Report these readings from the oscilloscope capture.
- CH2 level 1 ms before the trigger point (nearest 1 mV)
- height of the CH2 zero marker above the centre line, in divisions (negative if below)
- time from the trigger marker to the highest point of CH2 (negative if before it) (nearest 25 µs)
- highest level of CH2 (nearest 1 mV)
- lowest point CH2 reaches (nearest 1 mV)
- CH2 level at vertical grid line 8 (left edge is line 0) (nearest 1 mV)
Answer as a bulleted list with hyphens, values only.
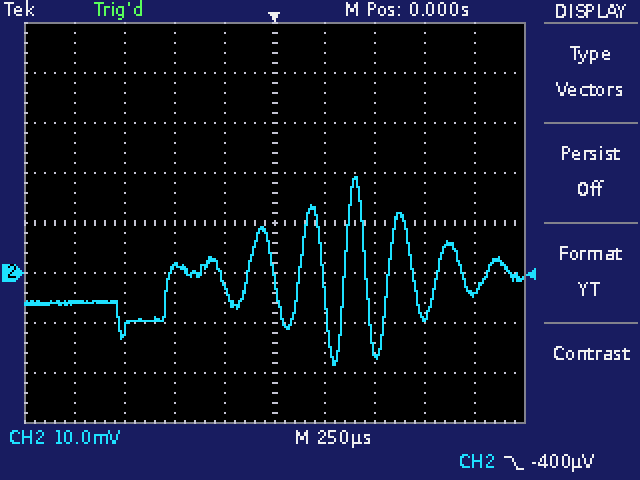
- -6 mV
- -1.0 div
- +400 µs
- 19 mV
- -18 mV
- -9 mV
